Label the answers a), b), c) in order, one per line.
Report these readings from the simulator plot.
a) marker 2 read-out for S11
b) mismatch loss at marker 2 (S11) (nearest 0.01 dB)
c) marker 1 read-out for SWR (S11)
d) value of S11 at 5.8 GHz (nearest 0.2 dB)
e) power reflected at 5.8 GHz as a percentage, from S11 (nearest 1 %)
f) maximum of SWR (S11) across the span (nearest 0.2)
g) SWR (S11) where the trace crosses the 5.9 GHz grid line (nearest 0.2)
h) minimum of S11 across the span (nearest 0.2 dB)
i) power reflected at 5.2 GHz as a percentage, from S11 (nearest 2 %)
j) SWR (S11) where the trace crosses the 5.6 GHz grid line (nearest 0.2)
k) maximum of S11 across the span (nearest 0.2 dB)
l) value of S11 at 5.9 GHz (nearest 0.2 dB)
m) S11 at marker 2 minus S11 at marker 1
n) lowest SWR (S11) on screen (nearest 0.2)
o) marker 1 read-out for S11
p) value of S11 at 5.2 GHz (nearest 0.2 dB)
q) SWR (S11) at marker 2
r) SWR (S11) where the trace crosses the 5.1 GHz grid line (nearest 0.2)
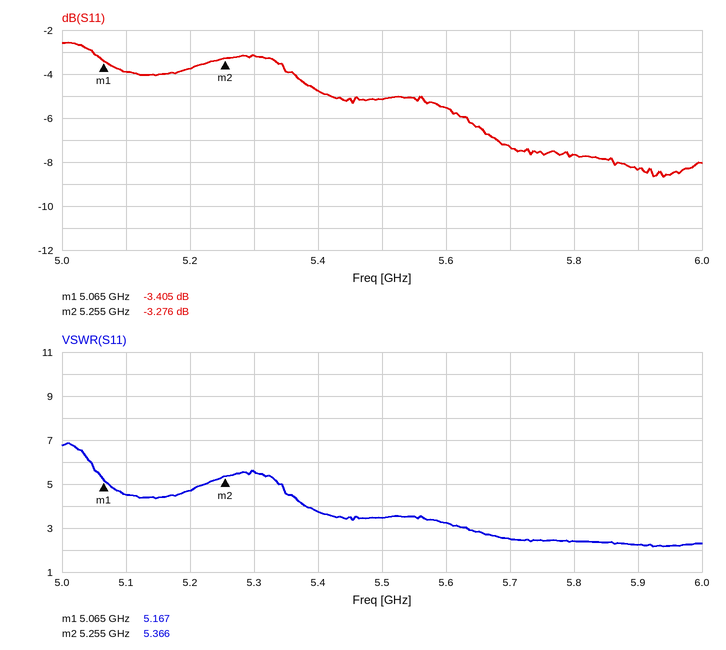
a) -3.276 dB
b) 2.76 dB
c) 5.167
d) -7.6 dB
e) 17 %
f) 6.8
g) 2.2
h) -8.6 dB
i) 42 %
j) 3.2
k) -2.6 dB
l) -8.4 dB
m) 0.129 dB
n) 2.2
o) -3.405 dB
p) -3.8 dB
q) 5.366
r) 4.6
